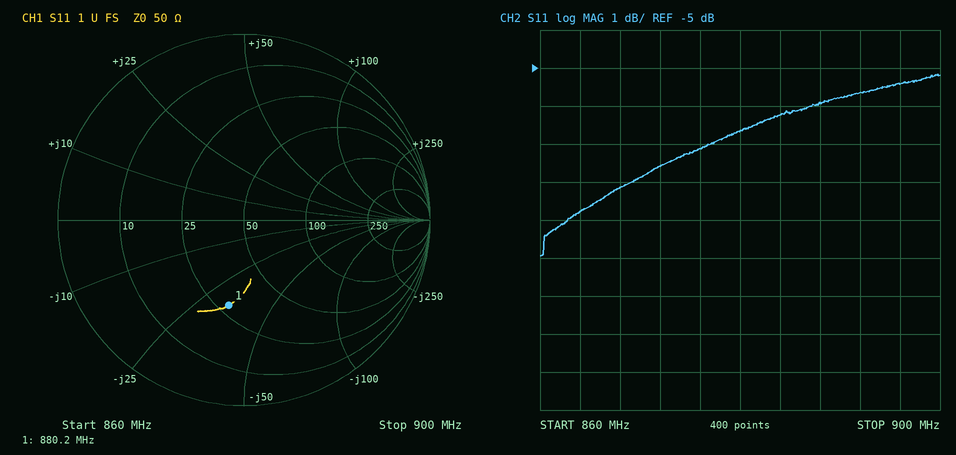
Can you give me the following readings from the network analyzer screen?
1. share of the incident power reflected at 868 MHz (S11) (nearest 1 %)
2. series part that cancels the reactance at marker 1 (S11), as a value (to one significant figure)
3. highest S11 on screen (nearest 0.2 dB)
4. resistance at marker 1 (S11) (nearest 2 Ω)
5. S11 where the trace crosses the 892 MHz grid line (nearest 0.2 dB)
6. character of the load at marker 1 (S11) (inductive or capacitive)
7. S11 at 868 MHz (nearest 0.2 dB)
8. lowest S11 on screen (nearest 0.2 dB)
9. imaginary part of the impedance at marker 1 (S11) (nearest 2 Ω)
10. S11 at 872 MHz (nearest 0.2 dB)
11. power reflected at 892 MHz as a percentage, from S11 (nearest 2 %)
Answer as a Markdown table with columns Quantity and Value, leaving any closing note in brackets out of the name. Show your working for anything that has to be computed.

| Quantity | Value |
|---|---|
| share of the incident power reflected at 868 MHz (S11) | 10^(-8.2/10) ≈ 15 % |
| series part that cancels the reactance at marker 1 (S11), as a value | L = 34 Ω/(2π × 880.2 MHz) ≈ 6 nH |
| highest S11 on screen | -5.2 dB |
| resistance at marker 1 (S11) | 28 Ω |
| S11 where the trace crosses the 892 MHz grid line | -5.6 dB |
| character of the load at marker 1 (S11) | capacitive |
| S11 at 868 MHz | -8.2 dB |
| lowest S11 on screen | -10.0 dB |
| imaginary part of the impedance at marker 1 (S11) | -34 Ω |
| S11 at 872 MHz | -7.6 dB |
| power reflected at 892 MHz as a percentage, from S11 | 10^(-5.6/10) ≈ 28 % |
